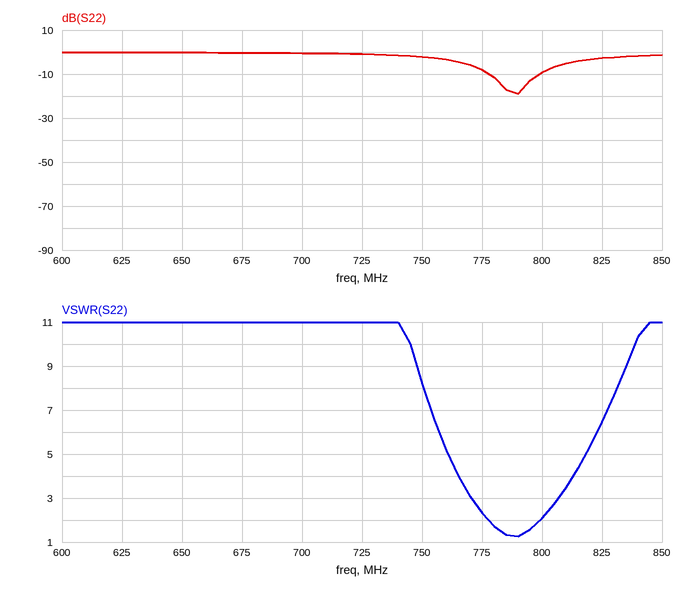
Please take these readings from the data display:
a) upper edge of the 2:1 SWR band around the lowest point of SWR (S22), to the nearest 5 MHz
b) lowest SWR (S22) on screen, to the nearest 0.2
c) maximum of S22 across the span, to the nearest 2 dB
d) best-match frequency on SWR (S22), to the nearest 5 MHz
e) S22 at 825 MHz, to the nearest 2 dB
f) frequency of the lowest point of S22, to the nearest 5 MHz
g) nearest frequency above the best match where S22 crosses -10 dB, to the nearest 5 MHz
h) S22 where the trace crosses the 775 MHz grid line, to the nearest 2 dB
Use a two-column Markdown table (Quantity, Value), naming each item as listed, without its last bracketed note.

| Quantity | Value |
|---|---|
| upper edge of the 2:1 SWR band around the lowest point of SWR (S22), to the nearest 5 MHz | 800 MHz |
| lowest SWR (S22) on screen, to the nearest 0.2 | 1.2 |
| maximum of S22 across the span, to the nearest 2 dB | 0 dB |
| best-match frequency on SWR (S22), to the nearest 5 MHz | 790 MHz |
| S22 at 825 MHz, to the nearest 2 dB | -2 dB |
| frequency of the lowest point of S22, to the nearest 5 MHz | 790 MHz |
| nearest frequency above the best match where S22 crosses -10 dB, to the nearest 5 MHz | 800 MHz |
| S22 where the trace crosses the 775 MHz grid line, to the nearest 2 dB | -8 dB |
